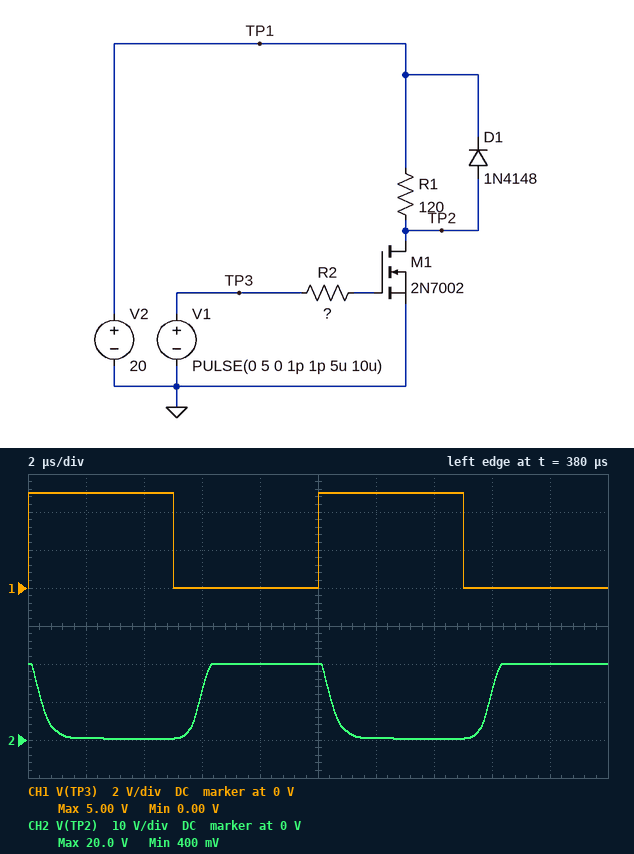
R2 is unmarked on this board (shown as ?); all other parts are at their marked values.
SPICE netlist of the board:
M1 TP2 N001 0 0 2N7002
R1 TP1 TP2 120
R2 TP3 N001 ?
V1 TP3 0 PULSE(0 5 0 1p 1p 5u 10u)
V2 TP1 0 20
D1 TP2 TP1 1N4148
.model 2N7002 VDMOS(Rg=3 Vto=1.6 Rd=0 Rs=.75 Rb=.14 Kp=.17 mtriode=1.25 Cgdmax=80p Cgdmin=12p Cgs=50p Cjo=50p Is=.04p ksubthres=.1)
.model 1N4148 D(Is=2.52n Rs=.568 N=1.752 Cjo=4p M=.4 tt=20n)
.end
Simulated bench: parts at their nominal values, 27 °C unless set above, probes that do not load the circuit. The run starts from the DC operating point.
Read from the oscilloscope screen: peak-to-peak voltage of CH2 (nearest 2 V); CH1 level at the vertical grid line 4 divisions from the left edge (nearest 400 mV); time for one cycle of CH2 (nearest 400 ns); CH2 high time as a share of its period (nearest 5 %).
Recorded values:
20 V
0 V
10.0 µs
45 %
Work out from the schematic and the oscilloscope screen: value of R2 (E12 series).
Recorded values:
4.7 kΩ
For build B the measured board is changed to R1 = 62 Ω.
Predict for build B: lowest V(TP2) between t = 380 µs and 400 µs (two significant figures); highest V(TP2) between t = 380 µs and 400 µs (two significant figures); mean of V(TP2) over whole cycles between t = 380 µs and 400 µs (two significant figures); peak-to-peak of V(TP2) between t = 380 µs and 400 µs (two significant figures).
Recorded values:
750 mV
20 V
10 V
19 V
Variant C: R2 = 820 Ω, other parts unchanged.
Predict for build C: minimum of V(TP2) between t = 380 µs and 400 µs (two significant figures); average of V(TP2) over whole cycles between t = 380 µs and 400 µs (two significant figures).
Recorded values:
360 mV
10 V
